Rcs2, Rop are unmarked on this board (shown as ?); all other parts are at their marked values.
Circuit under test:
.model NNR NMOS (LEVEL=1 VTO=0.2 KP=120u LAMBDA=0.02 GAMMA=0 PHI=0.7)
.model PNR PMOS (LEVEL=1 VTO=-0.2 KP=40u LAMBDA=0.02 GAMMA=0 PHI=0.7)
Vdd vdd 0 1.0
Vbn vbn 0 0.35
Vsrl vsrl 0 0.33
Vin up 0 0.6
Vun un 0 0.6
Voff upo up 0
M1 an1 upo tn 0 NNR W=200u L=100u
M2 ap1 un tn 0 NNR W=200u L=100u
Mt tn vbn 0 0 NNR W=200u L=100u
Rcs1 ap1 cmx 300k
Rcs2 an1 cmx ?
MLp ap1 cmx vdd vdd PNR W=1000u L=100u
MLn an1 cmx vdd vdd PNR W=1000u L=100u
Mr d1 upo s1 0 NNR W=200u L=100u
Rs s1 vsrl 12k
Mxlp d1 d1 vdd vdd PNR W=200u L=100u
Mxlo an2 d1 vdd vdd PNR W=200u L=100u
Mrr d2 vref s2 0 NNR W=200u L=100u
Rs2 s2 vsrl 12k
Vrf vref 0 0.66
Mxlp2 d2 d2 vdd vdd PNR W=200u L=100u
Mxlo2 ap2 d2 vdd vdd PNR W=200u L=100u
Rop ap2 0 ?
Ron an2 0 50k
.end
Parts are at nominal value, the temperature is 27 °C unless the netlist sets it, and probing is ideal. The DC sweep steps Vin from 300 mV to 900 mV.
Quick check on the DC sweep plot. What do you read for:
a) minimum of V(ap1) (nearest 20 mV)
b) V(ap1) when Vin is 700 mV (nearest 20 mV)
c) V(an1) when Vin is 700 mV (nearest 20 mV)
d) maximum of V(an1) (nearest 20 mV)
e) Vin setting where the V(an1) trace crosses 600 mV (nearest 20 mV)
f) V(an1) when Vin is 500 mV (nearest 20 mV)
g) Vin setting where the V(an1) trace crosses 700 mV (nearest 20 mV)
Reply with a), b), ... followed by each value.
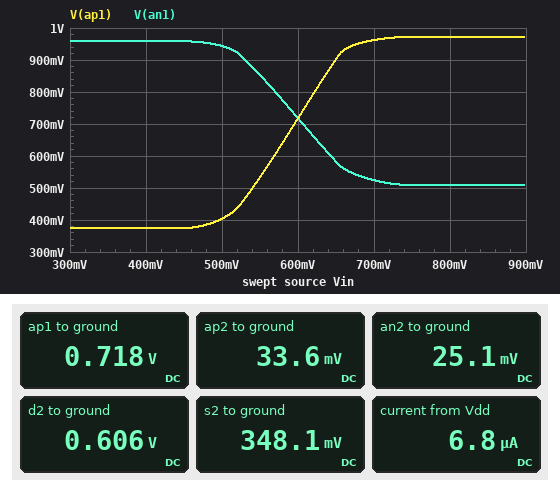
a) 380 mV
b) 960 mV
c) 520 mV
d) 960 mV
e) 640 mV
f) 940 mV
g) 600 mV
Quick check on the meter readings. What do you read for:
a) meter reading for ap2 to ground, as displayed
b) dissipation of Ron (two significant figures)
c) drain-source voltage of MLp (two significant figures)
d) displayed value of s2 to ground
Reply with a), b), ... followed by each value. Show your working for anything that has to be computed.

a) 33.6 mV
b) (25.1 mV)^2 / 50 kΩ = 13 nW
c) 718 mV - 1 V = -280 mV
d) 348.1 mV
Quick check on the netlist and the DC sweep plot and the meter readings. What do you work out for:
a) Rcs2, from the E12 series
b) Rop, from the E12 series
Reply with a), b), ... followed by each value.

a) 220 kΩ
b) 22 kΩ
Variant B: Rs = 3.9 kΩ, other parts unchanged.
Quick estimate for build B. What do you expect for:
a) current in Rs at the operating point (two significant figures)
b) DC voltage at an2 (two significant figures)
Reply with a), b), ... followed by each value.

a) 560 nA
b) 28 mV
